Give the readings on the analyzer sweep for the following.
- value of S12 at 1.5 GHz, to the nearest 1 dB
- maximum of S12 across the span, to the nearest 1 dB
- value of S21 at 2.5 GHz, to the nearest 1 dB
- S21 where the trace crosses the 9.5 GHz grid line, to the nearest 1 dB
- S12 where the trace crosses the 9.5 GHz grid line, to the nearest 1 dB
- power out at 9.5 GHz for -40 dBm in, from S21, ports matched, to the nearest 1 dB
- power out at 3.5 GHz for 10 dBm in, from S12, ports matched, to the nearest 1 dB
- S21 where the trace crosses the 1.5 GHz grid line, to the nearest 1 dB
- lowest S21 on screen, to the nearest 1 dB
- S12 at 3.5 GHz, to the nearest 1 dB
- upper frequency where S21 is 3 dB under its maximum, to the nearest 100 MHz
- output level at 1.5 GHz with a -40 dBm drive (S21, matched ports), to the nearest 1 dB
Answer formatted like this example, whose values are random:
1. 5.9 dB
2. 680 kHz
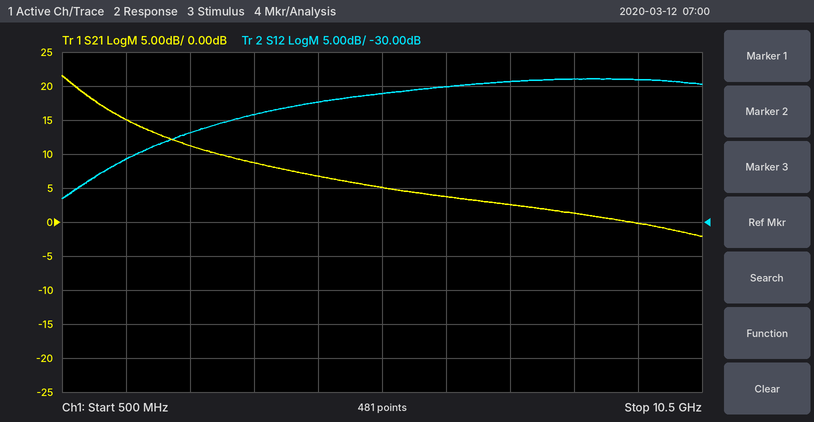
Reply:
1. -21 dB
2. -9 dB
3. 11 dB
4. 0 dB
5. -9 dB
6. -40 dBm
7. -4 dBm
8. 15 dB
9. -2 dB
10. -14 dB
11. 900 MHz
12. -25 dBm
